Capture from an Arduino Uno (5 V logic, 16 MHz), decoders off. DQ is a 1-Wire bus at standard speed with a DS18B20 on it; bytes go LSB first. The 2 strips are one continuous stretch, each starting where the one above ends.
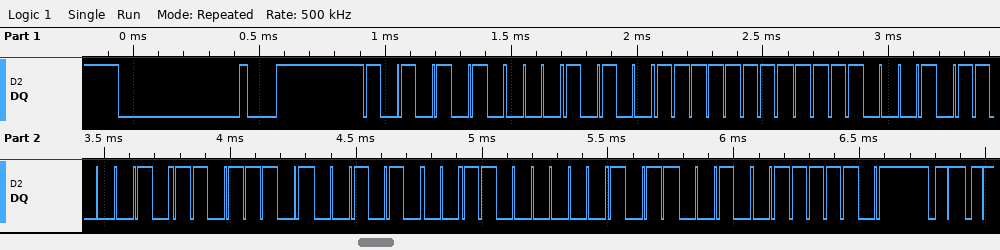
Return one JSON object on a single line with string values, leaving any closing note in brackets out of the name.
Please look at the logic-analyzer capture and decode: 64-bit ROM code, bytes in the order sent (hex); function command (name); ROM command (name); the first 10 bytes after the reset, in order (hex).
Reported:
{"64-bit ROM code, bytes in the order sent": "28 FF 8F 46 BB 14 03 4D", "function command": "Read Scratchpad", "ROM command": "Match ROM", "the first 10 bytes after the reset, in order": "55 28 FF 8F 46 BB 14 03 4D BE"}
